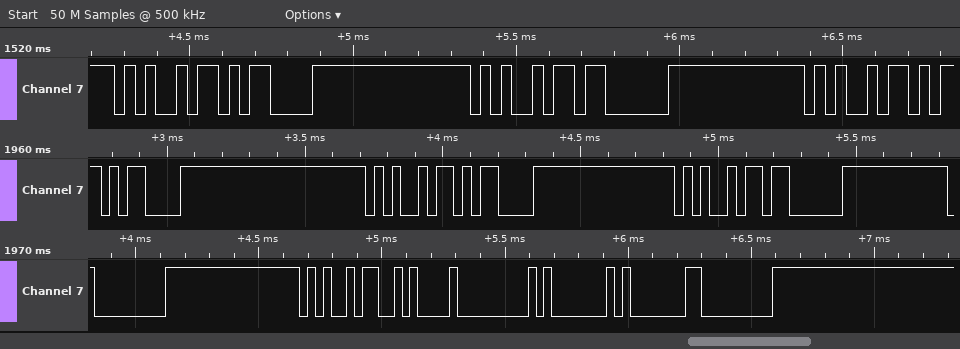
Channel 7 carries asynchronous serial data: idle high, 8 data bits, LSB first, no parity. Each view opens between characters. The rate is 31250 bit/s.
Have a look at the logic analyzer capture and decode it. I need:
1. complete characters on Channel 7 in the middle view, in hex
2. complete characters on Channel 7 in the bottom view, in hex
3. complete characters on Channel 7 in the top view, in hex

0D, A5, 0D, A5, 03
00, A5, 0A, 00, 01, 01, 00
A5, 0D, A5, 03, A5
